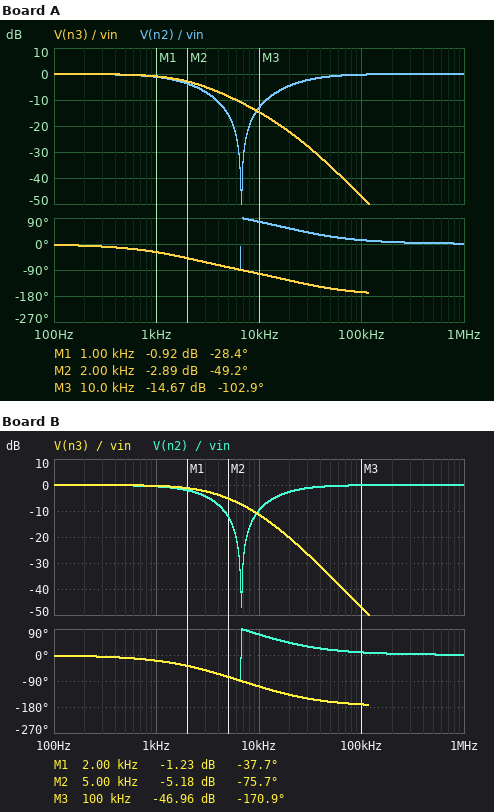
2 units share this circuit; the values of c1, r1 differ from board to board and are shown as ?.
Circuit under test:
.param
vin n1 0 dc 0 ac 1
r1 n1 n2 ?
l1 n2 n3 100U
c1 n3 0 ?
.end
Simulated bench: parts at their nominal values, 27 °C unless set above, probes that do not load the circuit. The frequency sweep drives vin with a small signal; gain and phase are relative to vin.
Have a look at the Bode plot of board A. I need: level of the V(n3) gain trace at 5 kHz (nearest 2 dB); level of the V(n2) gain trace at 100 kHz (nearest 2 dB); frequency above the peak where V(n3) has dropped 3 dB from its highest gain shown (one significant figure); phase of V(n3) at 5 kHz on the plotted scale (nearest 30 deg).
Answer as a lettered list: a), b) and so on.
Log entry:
a) -8 dB
b) 0 dB
c) 2 kHz
d) -90 deg
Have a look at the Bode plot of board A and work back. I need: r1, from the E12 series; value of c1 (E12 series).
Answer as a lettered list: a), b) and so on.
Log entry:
a) 15 Ω
b) 5.6 µF
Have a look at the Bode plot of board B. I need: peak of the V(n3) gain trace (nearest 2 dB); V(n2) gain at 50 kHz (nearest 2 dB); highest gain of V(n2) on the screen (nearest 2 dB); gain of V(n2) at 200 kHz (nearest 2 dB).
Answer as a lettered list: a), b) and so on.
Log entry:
a) 0 dB
b) 0 dB
c) 0 dB
d) 0 dB
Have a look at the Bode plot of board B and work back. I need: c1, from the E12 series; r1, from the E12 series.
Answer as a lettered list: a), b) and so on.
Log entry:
a) 5.6 µF
b) 10 Ω
